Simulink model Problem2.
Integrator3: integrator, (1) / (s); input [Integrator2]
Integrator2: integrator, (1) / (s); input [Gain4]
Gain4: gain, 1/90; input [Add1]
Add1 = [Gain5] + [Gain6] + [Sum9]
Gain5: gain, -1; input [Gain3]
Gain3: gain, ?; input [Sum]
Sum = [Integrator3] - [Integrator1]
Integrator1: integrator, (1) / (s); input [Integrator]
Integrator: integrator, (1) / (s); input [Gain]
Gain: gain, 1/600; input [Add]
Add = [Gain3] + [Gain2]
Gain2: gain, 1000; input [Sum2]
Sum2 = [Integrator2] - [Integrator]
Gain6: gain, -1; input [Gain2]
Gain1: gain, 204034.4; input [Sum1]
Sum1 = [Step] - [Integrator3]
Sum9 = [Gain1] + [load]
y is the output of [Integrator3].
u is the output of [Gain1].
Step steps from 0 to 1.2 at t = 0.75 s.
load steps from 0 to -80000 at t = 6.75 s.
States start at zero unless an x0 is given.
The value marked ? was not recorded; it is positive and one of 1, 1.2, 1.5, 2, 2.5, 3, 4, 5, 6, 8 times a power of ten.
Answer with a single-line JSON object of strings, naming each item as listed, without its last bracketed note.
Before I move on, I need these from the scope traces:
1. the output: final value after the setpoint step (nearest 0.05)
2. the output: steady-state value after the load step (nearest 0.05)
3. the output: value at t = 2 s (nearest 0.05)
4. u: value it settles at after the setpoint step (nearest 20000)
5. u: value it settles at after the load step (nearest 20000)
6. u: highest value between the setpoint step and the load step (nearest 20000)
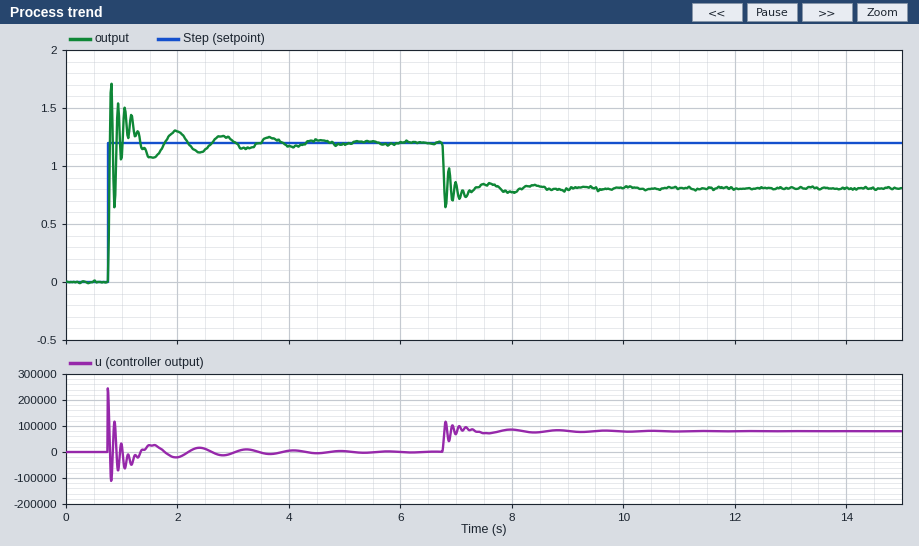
{"the output: final value after the setpoint step": "1.20", "the output: steady-state value after the load step": "0.80", "the output: value at t = 2 s": "1.30", "u: value it settles at after the setpoint step": "0", "u: value it settles at after the load step": "80000", "u: highest value between the setpoint step and the load step": "240000"}
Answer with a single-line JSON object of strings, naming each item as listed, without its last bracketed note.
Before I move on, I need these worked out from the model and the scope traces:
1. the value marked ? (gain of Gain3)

{"the value marked ?": "40000"}
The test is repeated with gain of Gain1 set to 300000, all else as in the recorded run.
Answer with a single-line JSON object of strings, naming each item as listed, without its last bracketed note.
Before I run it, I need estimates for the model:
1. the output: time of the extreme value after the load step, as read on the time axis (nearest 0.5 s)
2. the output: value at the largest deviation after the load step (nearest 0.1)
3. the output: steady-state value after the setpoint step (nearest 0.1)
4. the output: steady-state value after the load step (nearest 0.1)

{"the output: time of the extreme value after the load step, as read on the time axis": "7.0 s", "the output: value at the largest deviation after the load step": "0.8", "the output: steady-state value after the setpoint step": "1.2", "the output: steady-state value after the load step": "0.9"}
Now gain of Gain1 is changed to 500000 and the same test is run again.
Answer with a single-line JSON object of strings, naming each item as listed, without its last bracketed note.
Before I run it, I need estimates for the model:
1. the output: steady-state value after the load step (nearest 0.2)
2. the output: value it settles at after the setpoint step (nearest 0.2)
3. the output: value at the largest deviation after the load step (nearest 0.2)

{"the output: steady-state value after the load step": "1.0", "the output: value it settles at after the setpoint step": "1.2", "the output: value at the largest deviation after the load step": "1.0"}
